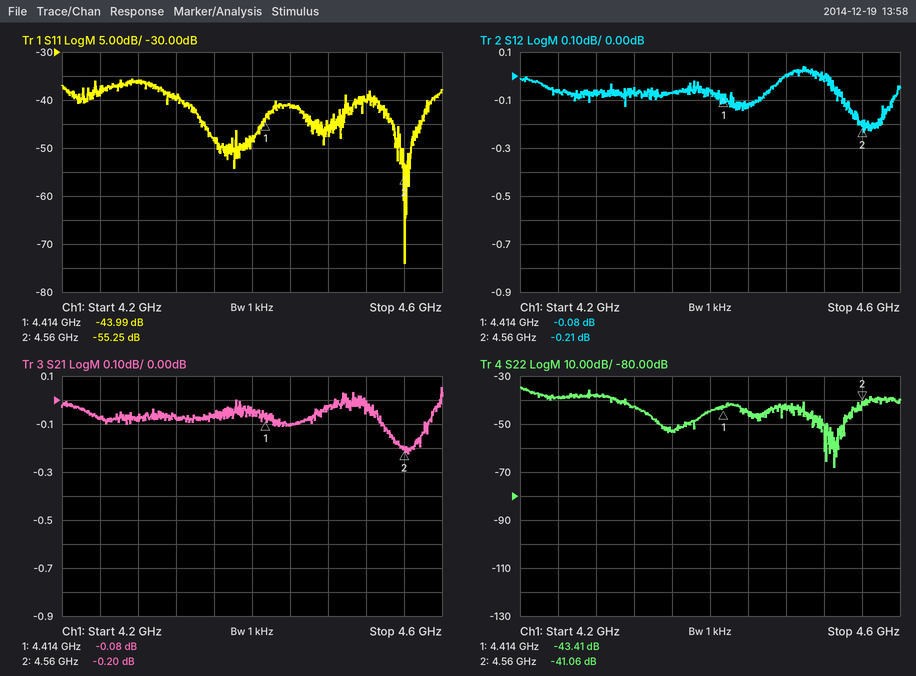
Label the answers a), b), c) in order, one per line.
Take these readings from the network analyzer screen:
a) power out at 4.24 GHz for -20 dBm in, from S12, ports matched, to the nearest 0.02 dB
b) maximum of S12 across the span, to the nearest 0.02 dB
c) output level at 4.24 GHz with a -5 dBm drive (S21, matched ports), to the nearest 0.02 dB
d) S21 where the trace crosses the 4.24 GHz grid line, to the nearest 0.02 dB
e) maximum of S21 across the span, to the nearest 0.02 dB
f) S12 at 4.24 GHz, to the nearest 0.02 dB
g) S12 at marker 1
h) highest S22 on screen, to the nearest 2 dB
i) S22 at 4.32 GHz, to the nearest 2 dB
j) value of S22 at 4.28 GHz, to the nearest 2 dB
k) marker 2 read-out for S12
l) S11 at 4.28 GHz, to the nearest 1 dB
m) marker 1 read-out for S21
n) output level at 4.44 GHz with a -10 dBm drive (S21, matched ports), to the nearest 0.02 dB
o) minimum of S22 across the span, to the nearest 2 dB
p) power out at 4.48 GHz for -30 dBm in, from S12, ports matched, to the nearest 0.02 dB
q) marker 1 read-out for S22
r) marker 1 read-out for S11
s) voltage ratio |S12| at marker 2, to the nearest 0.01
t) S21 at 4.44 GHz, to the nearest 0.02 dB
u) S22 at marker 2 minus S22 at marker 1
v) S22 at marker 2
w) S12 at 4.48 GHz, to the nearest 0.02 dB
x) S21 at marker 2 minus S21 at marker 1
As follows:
a) -20.06 dBm
b) 0.04 dB
c) -5.08 dBm
d) -0.08 dB
e) 0.06 dB
f) -0.06 dB
g) -0.08 dB
h) -34 dB
i) -42 dB
j) -38 dB
k) -0.21 dB
l) -36 dB
m) -0.08 dB
n) -10.10 dBm
o) -68 dB
p) -30.00 dBm
q) -43.41 dB
r) -43.99 dB
s) 0.98
t) -0.10 dB
u) 2.35 dB
v) -41.06 dB
w) 0.00 dB
x) -0.12 dB
